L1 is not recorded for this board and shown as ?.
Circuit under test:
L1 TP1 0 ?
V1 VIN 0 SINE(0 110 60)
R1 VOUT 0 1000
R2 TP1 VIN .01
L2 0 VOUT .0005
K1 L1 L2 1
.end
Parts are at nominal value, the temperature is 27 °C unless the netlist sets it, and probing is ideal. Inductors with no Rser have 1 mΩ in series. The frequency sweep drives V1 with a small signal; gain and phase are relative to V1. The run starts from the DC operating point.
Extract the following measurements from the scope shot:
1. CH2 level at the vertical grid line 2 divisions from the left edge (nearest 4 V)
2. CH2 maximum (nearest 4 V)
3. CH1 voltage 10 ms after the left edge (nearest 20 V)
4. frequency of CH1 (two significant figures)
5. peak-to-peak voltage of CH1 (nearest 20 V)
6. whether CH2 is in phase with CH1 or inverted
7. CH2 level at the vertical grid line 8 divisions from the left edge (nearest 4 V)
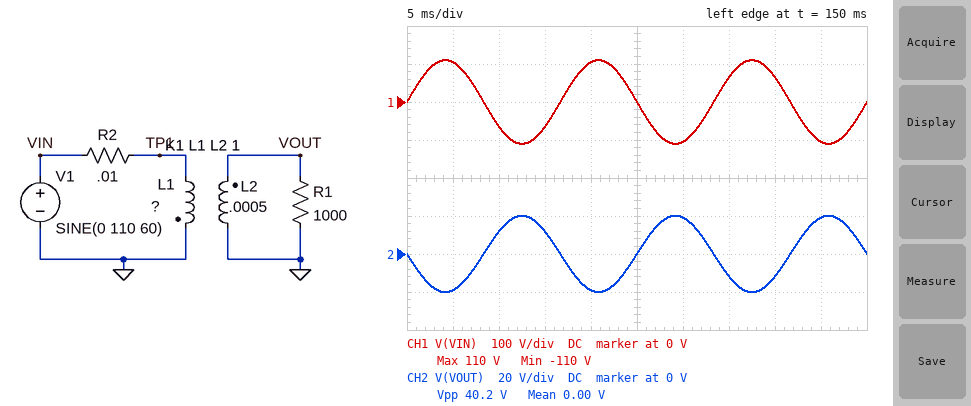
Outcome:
12 V
20 V
-60 V
60 Hz
220 V
inverted
-12 V
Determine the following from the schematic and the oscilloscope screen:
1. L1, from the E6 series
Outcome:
15 mH
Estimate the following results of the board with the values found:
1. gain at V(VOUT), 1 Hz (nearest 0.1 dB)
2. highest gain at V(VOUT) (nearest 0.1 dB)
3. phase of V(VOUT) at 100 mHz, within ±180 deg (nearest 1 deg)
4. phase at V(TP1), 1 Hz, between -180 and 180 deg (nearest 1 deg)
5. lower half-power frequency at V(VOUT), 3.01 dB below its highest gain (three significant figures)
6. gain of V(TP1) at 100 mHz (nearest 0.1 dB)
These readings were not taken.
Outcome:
-14.8 dB
-14.8 dB
-131 deg
6 deg
117 mHz
-3.7 dB
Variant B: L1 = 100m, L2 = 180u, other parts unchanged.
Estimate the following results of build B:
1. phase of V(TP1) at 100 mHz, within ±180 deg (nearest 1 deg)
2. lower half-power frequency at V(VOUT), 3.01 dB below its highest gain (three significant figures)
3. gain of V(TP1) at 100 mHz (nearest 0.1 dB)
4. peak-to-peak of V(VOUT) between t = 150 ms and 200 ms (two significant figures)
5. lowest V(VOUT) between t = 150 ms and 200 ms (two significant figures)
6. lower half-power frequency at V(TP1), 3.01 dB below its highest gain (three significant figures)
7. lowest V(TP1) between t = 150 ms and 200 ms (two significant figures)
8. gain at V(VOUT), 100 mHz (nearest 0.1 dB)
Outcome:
9 deg
17.5 mHz
-0.1 dB
9.3 V
-4.7 V
17.4 mHz
-110 V
-27.6 dB
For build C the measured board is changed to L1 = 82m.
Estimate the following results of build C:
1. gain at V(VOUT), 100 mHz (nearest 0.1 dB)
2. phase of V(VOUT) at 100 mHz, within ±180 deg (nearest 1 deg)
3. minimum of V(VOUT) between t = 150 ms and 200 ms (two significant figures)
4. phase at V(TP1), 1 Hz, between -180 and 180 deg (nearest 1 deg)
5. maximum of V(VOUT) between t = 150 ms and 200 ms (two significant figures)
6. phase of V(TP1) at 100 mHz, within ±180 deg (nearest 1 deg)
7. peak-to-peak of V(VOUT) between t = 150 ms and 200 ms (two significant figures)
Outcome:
-22.3 dB
-168 deg
-8.6 V
1 deg
8.6 V
11 deg
17 V
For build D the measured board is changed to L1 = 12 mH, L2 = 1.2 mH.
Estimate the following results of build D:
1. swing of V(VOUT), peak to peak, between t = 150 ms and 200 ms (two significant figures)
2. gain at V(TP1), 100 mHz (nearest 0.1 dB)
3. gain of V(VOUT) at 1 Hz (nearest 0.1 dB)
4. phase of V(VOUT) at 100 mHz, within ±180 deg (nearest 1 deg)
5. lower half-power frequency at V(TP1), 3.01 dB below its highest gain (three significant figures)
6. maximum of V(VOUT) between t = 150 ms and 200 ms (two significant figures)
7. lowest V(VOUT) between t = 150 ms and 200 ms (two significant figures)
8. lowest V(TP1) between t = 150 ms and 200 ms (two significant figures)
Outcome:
70 V
-4.9 dB
-10.1 dB
-124 deg
145 mHz
35 V
-35 V
-110 V
